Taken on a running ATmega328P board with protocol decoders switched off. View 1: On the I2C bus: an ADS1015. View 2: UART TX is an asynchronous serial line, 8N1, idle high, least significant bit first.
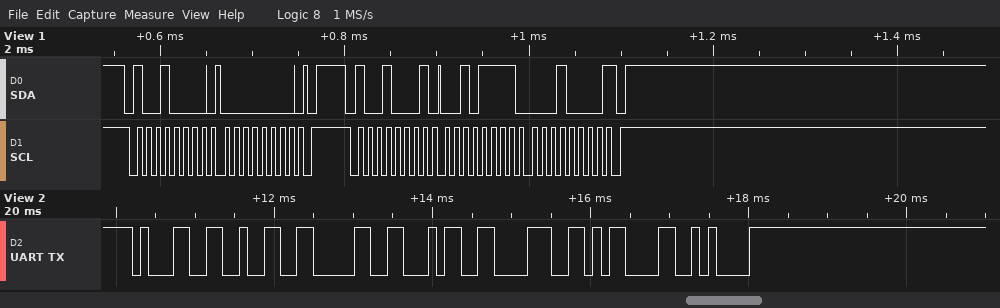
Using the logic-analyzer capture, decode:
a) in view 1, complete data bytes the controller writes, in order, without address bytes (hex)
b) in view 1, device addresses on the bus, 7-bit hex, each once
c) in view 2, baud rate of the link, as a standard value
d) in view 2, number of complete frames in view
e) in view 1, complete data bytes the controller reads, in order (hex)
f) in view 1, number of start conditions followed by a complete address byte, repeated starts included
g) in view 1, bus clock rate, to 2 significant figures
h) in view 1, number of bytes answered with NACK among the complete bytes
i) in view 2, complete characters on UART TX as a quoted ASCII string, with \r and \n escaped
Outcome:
00
0x48
9600 baud
7
2F 10
2
100 kHz
1
"12048\r\n"
